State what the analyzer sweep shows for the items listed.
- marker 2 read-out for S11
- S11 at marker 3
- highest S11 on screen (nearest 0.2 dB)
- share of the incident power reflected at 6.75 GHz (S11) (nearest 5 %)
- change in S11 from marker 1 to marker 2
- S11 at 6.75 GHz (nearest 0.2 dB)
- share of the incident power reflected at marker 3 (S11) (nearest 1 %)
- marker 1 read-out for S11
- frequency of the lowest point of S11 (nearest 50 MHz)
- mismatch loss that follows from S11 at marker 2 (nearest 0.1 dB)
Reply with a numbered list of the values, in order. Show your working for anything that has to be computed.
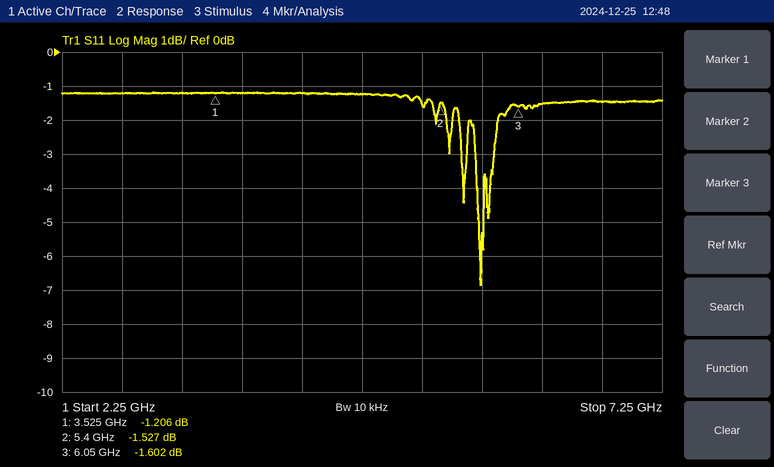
1. -1.527 dB
2. -1.602 dB
3. -1.2 dB
4. 10^(-1.4/10) ≈ 72.4 %, so 70 % to the nearest 5 %
5. -1.527 − (-1.206) = -0.321 dB
6. -1.4 dB
7. 10^(-1.602/10) ≈ 69 %
8. -1.206 dB
9. 5.75 GHz
10. −10 log10(1 − 10^(-1.527/10)) ≈ 5.3 dB
